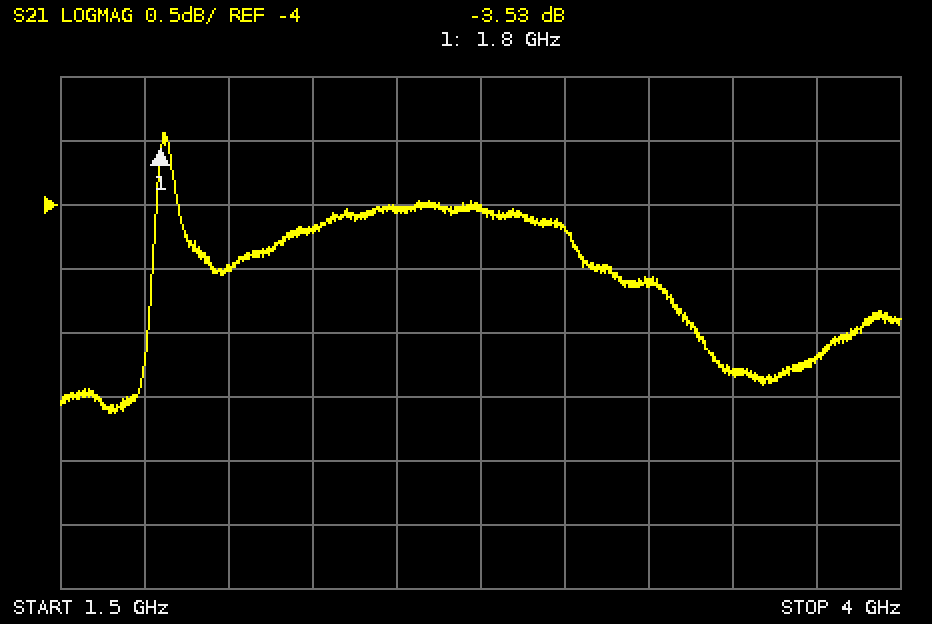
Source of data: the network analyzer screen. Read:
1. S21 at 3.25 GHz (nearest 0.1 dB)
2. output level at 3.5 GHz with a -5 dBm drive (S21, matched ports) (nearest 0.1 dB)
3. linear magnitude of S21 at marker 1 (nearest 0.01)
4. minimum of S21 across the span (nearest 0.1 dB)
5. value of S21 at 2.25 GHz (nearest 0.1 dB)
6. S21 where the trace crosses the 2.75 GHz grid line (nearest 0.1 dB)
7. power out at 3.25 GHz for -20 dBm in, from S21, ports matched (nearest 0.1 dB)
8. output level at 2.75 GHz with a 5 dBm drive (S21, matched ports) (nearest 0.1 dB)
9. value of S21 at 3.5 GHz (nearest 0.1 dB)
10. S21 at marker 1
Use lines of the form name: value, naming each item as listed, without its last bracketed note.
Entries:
S21 at 3.25 GHz: -4.6 dB
output level at 3.5 GHz with a -5 dBm drive (S21, matched ports): -10.3 dBm
linear magnitude of S21 at marker 1: 0.67
minimum of S21 across the span: -5.6 dB
value of S21 at 2.25 GHz: -4.2 dB
S21 where the trace crosses the 2.75 GHz grid line: -4.0 dB
power out at 3.25 GHz for -20 dBm in, from S21, ports matched: -24.6 dBm
output level at 2.75 GHz with a 5 dBm drive (S21, matched ports): 1.0 dBm
value of S21 at 3.5 GHz: -5.3 dB
S21 at marker 1: -3.53 dB
